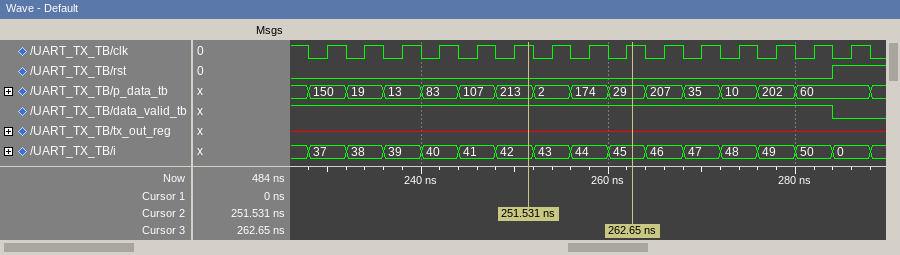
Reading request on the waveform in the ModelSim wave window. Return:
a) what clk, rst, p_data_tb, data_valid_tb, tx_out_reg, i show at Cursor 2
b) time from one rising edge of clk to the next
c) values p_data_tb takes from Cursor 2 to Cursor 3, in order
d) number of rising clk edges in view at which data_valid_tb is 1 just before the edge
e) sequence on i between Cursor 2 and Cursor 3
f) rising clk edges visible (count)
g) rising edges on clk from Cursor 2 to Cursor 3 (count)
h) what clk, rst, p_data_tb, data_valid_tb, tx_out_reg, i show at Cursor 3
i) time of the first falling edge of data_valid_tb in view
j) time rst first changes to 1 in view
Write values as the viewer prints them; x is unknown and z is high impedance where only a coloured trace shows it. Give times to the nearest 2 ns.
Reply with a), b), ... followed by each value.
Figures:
a) clk=1, rst=0, p_data_tb=213, data_valid_tb=1, tx_out_reg=x, i=42
b) 4 ns
c) 213, 2, 174, 29
d) 14
e) 42, 43, 44, 45
f) 15
g) 3
h) clk=1, rst=0, p_data_tb=29, data_valid_tb=1, tx_out_reg=x, i=45
i) 284 ns
j) 284 ns
